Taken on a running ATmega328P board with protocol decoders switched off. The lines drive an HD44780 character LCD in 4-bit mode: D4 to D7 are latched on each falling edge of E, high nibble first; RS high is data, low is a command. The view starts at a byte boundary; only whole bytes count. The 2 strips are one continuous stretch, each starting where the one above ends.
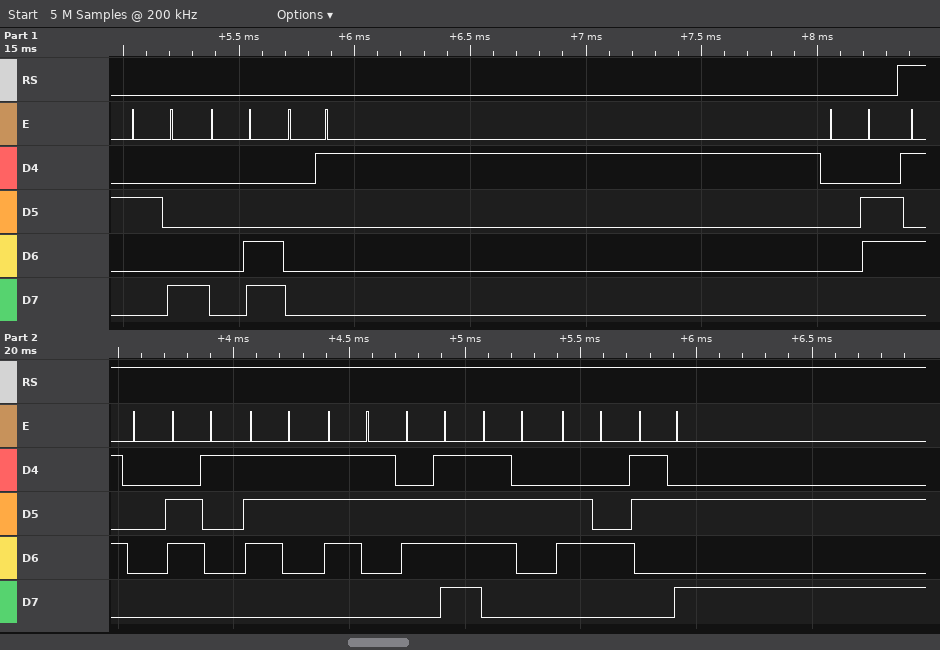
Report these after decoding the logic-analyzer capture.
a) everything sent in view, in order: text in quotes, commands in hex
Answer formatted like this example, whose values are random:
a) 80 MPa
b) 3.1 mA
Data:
a) 0x28 0x0C 0x01 0x06 "Passord:"
